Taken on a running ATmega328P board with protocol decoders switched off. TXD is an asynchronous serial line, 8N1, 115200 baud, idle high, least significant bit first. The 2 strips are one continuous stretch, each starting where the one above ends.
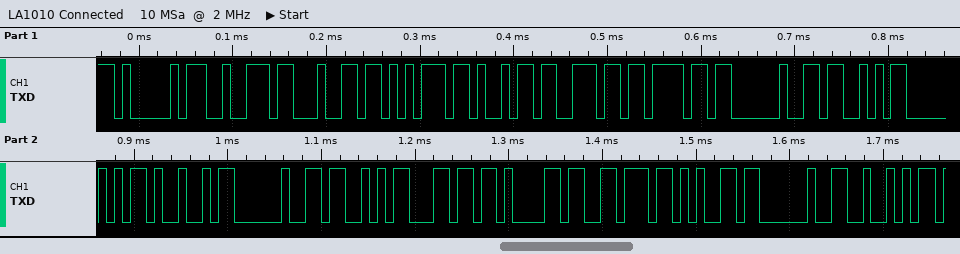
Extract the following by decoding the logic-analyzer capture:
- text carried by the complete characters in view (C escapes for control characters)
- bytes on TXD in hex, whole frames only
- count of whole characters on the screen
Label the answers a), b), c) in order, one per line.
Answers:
a) "Arduino SPI Slave R"
b) 41 72 64 75 69 6E 6F 20 53 50 49 20 53 6C 61 76 65 20 52
c) 19
